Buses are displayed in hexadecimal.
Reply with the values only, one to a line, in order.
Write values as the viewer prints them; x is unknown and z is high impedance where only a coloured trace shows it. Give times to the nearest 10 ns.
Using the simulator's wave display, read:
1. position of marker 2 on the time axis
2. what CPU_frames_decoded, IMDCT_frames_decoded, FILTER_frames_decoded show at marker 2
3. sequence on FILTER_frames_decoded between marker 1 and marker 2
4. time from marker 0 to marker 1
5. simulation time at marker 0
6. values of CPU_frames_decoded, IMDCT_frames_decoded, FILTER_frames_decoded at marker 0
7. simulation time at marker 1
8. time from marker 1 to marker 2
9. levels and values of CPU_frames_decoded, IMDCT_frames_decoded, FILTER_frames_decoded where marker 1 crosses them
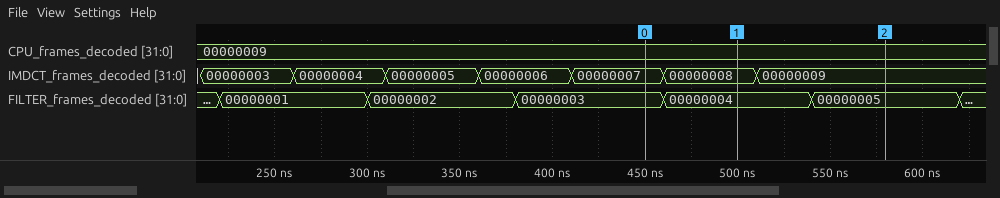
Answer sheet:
580 ns
CPU_frames_decoded=00000009, IMDCT_frames_decoded=00000009, FILTER_frames_decoded=00000005
00000004, 00000005
50 ns
450 ns
CPU_frames_decoded=00000009, IMDCT_frames_decoded=00000007, FILTER_frames_decoded=00000003
500 ns
80 ns
CPU_frames_decoded=00000009, IMDCT_frames_decoded=00000008, FILTER_frames_decoded=00000004
